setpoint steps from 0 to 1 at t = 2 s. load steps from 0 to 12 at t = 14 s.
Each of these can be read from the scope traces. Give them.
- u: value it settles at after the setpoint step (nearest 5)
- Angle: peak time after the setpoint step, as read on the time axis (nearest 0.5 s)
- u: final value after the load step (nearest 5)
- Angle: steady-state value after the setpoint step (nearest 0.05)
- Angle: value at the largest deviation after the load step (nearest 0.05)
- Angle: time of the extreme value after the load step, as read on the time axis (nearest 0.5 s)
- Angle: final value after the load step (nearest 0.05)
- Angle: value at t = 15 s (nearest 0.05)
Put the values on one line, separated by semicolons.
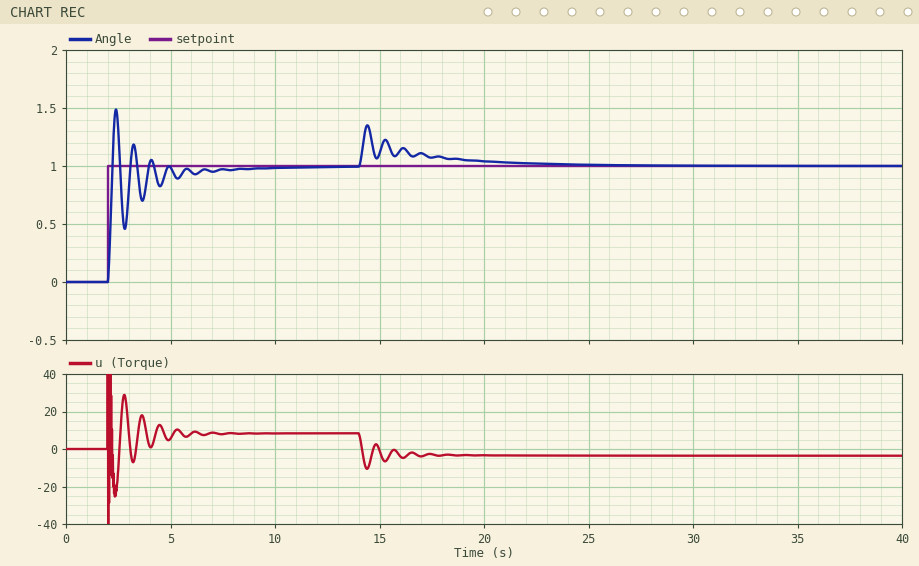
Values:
10; 2.5 s; -5; 1.00; 1.35; 14.5 s; 1.00; 1.10
